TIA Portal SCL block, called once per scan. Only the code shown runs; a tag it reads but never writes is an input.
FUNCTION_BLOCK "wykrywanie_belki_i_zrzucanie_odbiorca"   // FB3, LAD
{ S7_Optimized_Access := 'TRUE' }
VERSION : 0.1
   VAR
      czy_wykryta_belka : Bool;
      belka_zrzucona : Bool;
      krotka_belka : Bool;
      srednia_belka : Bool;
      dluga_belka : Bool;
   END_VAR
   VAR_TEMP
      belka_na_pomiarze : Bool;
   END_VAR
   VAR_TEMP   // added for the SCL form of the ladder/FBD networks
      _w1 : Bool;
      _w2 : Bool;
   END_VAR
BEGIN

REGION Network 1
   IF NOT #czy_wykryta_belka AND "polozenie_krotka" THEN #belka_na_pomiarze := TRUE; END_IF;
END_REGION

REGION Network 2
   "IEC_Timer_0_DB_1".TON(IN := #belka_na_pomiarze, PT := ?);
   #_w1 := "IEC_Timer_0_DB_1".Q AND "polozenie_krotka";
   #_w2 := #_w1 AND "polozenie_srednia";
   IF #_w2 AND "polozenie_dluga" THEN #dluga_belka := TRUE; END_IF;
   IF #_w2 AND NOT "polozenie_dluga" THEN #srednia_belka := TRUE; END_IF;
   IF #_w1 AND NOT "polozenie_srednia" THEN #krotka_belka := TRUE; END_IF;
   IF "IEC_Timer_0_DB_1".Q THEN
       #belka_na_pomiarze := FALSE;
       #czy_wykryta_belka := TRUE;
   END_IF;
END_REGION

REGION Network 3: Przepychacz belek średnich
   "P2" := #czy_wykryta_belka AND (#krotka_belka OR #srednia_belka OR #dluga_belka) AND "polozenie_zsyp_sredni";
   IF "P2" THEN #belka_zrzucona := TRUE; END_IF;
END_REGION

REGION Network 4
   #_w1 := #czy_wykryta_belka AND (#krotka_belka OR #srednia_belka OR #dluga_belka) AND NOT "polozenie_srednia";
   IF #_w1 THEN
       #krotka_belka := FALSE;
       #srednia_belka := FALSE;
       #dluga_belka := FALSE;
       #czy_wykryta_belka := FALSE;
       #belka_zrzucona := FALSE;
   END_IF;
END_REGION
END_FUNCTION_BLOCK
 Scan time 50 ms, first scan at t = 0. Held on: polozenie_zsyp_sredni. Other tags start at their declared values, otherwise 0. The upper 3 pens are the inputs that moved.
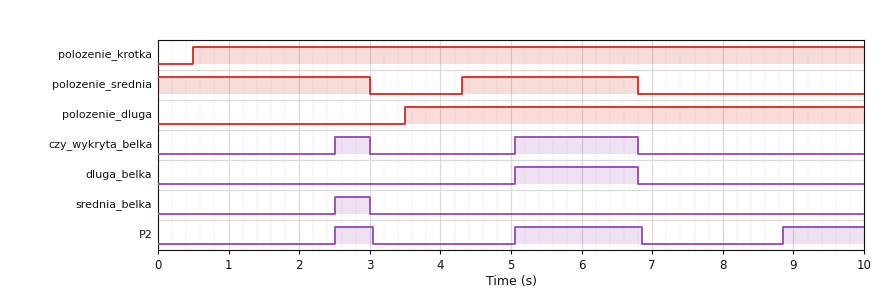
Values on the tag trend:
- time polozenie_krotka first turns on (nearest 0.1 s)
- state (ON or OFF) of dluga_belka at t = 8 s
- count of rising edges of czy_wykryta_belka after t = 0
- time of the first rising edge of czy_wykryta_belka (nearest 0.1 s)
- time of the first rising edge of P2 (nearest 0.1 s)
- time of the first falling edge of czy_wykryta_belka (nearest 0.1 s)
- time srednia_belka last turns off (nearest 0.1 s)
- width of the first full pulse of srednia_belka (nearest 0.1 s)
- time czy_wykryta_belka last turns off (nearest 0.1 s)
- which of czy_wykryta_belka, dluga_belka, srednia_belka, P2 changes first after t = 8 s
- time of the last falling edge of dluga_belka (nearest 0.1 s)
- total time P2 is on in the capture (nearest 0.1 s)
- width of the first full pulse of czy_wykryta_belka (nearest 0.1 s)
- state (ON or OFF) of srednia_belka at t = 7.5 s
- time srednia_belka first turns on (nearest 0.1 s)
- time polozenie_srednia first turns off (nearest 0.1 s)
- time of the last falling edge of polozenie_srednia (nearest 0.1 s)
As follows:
0.5 s
OFF
2
2.5 s
2.5 s
3.0 s
3.0 s
0.5 s
6.8 s
P2
6.8 s
3.5 s
0.5 s
OFF
2.5 s
3.0 s
6.8 s
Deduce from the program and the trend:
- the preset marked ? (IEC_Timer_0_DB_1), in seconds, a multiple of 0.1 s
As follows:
2.0 s
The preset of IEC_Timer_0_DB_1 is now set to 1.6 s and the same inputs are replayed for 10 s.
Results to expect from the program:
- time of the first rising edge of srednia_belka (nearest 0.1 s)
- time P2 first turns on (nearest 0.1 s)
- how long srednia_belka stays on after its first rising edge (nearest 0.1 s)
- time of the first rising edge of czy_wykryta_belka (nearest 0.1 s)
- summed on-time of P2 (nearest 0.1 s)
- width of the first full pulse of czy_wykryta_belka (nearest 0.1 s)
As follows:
2.1 s
2.1 s
0.9 s
2.1 s
4.7 s
0.9 s
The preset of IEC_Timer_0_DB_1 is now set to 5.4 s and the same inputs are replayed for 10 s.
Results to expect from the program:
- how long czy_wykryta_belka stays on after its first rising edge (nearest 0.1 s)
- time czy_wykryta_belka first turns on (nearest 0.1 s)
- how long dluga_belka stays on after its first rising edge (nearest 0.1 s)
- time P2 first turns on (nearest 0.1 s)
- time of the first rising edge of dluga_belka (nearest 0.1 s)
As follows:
0.9 s
5.9 s
0.9 s
5.9 s
5.9 s
